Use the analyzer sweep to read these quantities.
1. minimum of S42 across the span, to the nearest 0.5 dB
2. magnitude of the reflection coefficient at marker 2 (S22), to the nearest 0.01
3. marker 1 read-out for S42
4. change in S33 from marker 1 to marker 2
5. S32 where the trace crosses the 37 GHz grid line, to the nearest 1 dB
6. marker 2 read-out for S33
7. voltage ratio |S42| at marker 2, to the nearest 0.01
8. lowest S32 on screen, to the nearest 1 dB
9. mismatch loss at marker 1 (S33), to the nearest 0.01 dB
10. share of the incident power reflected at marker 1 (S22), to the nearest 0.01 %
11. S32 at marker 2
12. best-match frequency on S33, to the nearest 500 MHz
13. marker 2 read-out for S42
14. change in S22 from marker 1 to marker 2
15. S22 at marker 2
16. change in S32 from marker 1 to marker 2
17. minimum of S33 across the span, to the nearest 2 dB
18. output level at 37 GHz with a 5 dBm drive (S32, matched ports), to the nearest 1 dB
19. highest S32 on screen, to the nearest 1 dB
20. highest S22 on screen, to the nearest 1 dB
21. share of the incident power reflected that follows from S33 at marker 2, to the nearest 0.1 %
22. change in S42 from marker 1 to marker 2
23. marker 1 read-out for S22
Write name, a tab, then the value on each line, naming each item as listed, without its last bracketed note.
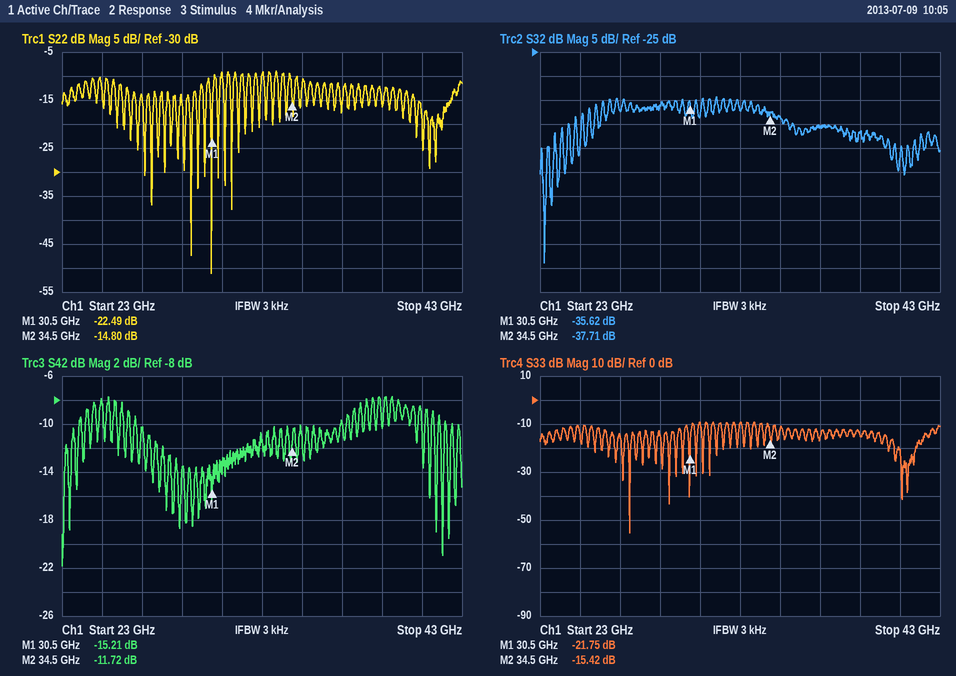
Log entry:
minimum of S42 across the span, to the nearest 0.5 dB	-22.0 dB
magnitude of the reflection coefficient at marker 2 (S22), to the nearest 0.01	0.18
marker 1 read-out for S42	-15.21 dB
change in S33 from marker 1 to marker 2	6.33 dB
S32 where the trace crosses the 37 GHz grid line, to the nearest 1 dB	-41 dB
marker 2 read-out for S33	-15.42 dB
voltage ratio |S42| at marker 2, to the nearest 0.01	0.26
lowest S32 on screen, to the nearest 1 dB	-69 dB
mismatch loss at marker 1 (S33), to the nearest 0.01 dB	0.03 dB
share of the incident power reflected at marker 1 (S22), to the nearest 0.01 %	0.56 %
S32 at marker 2	-37.71 dB
best-match frequency on S33, to the nearest 500 MHz	27.5 GHz
marker 2 read-out for S42	-11.72 dB
change in S22 from marker 1 to marker 2	7.69 dB
S22 at marker 2	-14.80 dB
change in S32 from marker 1 to marker 2	-2.09 dB
minimum of S33 across the span, to the nearest 2 dB	-56 dB
output level at 37 GHz with a 5 dBm drive (S32, matched ports), to the nearest 1 dB	-36 dBm
highest S32 on screen, to the nearest 1 dB	-34 dB
highest S22 on screen, to the nearest 1 dB	-9 dB
share of the incident power reflected that follows from S33 at marker 2, to the nearest 0.1 %	2.9 %
change in S42 from marker 1 to marker 2	3.49 dB
marker 1 read-out for S22	-22.49 dB
